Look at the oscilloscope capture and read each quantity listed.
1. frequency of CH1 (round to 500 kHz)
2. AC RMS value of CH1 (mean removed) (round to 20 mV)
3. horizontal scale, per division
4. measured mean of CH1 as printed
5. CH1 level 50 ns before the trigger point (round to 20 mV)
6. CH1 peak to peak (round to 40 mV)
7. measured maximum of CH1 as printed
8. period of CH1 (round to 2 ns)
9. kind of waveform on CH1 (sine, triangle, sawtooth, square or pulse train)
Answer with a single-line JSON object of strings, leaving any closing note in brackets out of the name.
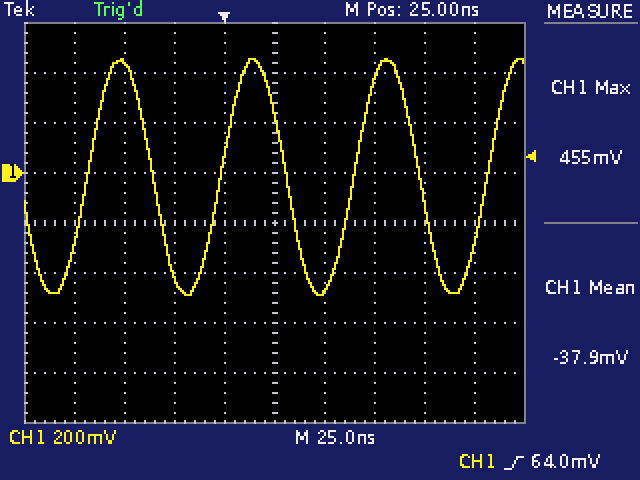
{"frequency of CH1": "15.0 MHz", "AC RMS value of CH1 (mean removed)": "340 mV", "horizontal scale, per division": "25 ns", "measured mean of CH1 as printed": "-37.9 mV", "CH1 level 50 ns before the trigger point": "440 mV", "CH1 peak to peak": "960 mV", "measured maximum of CH1 as printed": "455 mV", "period of CH1": "66 ns", "kind of waveform on CH1": "sine"}
